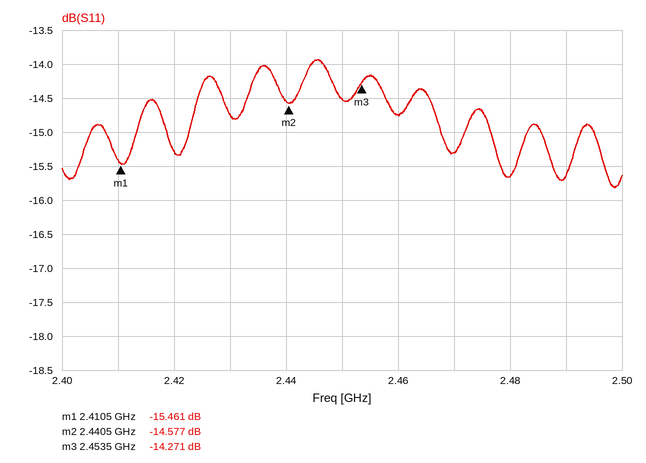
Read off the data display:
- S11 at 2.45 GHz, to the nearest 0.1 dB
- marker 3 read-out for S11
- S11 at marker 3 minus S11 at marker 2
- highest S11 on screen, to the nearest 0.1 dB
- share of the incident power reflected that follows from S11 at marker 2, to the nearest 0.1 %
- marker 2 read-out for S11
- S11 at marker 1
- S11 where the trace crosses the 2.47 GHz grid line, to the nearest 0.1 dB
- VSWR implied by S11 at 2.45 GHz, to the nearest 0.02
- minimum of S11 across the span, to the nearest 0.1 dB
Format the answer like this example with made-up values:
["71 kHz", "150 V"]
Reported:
["-14.5 dB", "-14.271 dB", "0.306 dB", "-13.9 dB", "3.5 %", "-14.577 dB", "-15.461 dB", "-15.3 dB", "1.46", "-15.8 dB"]
